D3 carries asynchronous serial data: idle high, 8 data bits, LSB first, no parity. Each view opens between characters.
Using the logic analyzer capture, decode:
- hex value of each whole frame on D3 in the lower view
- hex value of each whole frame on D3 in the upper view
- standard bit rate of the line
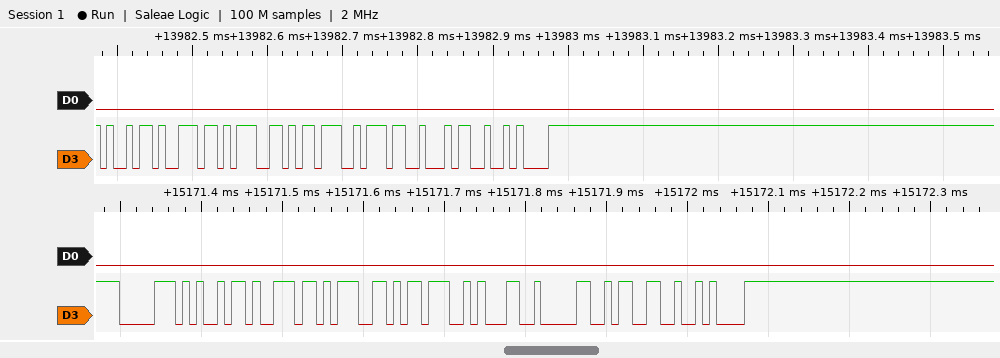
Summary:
70, 69, 6E, 67, 3B, 31, 30, 33, 0A
69, 6E, 67, 3B, 37, 34, 0A
115200 baud
